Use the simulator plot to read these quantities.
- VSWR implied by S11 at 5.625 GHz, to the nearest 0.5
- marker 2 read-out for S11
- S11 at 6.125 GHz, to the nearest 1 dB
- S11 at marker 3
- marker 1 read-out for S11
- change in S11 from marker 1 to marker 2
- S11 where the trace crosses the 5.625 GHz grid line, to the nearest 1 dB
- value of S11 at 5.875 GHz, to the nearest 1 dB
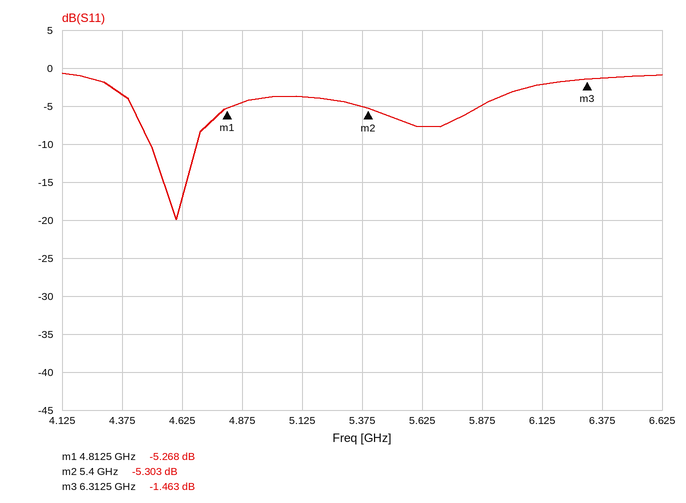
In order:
2.5
-5.303 dB
-2 dB
-1.463 dB
-5.268 dB
-0.035 dB
-8 dB
-5 dB
